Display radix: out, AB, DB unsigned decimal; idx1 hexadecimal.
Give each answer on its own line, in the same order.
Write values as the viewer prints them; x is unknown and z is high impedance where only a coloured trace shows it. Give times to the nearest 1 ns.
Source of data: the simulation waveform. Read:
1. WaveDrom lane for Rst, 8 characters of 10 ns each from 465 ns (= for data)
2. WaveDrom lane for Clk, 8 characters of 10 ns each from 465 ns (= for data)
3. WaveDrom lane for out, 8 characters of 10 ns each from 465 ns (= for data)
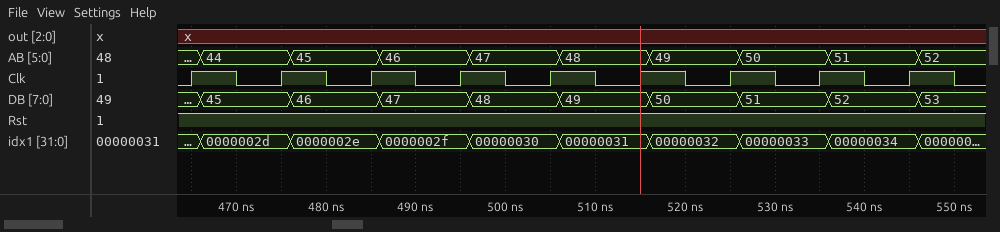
{name: 'Rst', wave: '1.......'}
{name: 'Clk', wave: 'p.......'}
{name: 'out', wave: 'x.......'}
